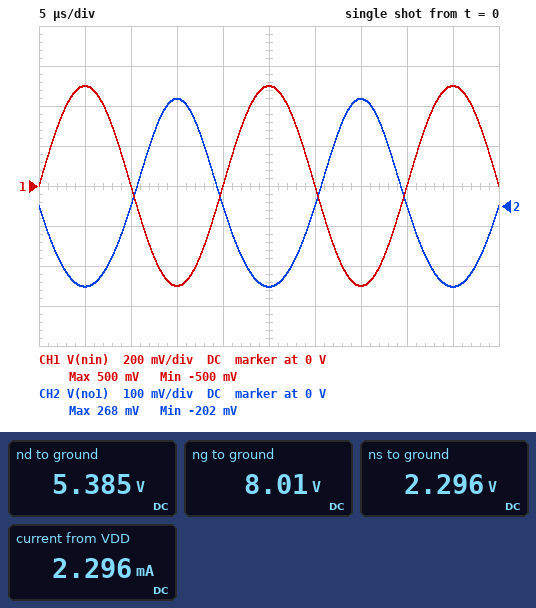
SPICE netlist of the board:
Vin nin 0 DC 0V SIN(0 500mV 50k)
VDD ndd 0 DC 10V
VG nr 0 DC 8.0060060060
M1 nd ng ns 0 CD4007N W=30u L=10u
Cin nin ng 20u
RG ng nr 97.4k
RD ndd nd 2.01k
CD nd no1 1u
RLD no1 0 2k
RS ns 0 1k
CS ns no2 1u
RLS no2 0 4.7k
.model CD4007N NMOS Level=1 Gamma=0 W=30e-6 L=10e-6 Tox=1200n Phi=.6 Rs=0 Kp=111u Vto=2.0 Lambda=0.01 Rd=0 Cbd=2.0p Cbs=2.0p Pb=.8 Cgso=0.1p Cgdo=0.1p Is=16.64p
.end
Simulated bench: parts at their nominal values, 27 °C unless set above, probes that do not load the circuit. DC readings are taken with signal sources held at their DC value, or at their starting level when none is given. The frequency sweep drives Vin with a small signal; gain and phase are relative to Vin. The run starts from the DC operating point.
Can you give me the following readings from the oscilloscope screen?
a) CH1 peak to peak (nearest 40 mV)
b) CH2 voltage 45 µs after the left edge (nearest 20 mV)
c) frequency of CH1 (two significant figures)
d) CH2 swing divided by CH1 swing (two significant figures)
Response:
1.00 V
-200 mV
50 kHz
0.47
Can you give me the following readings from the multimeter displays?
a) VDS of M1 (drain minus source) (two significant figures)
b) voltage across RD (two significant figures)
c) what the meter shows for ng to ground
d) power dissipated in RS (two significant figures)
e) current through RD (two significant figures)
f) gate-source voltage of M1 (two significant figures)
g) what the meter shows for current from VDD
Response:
3.1 V
4.6 V
8.01 V
5.3 mW
2.3 mA
5.7 V
2.296 mA
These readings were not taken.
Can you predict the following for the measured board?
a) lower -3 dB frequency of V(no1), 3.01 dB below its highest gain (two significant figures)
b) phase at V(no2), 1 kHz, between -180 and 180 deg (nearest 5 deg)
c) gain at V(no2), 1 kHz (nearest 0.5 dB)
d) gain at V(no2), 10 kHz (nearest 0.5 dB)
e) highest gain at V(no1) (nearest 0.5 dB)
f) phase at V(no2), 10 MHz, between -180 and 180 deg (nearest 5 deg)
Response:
46 Hz
0 deg
-8.5 dB
-8.5 dB
-6.5 dB
0 deg
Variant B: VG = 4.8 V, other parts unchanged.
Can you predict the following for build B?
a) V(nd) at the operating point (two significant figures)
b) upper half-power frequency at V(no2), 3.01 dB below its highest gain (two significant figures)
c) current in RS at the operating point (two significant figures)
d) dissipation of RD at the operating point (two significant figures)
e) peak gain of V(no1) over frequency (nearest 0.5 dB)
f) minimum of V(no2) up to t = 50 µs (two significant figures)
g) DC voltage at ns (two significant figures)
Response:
8.5 V
220 MHz
750 µA
1.1 mW
-6.0 dB
-180 mV
750 mV
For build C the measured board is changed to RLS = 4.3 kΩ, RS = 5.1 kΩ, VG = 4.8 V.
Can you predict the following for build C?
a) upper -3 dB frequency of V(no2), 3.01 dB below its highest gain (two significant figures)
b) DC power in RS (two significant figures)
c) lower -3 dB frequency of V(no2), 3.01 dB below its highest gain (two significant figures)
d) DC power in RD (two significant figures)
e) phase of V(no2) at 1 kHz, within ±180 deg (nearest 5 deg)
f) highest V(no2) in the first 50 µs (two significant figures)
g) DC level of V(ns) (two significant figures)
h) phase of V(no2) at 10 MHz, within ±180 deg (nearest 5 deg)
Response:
120 MHz
450 µW
27 Hz
180 µW
0 deg
270 mV
1.5 V
-5 deg
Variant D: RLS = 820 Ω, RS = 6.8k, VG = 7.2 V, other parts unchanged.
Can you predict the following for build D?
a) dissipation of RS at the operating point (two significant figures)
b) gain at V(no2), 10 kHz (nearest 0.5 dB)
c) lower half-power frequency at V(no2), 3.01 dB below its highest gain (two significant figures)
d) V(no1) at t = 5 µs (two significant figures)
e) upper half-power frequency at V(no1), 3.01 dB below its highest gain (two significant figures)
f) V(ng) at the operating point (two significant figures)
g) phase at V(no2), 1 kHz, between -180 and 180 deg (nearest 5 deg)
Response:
1.8 mW
-10.5 dB
74 Hz
-220 mV
410 MHz
7.2 V
5 deg
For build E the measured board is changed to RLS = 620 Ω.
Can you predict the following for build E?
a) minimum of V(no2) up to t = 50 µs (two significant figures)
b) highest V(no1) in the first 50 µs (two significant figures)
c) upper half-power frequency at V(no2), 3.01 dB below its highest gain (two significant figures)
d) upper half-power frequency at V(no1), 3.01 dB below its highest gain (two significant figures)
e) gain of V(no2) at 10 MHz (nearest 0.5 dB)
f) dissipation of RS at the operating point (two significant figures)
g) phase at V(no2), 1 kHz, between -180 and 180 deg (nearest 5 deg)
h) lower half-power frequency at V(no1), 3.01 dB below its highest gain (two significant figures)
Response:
-140 mV
360 mV
750 MHz
300 MHz
-12.5 dB
5.3 mW
10 deg
92 Hz
